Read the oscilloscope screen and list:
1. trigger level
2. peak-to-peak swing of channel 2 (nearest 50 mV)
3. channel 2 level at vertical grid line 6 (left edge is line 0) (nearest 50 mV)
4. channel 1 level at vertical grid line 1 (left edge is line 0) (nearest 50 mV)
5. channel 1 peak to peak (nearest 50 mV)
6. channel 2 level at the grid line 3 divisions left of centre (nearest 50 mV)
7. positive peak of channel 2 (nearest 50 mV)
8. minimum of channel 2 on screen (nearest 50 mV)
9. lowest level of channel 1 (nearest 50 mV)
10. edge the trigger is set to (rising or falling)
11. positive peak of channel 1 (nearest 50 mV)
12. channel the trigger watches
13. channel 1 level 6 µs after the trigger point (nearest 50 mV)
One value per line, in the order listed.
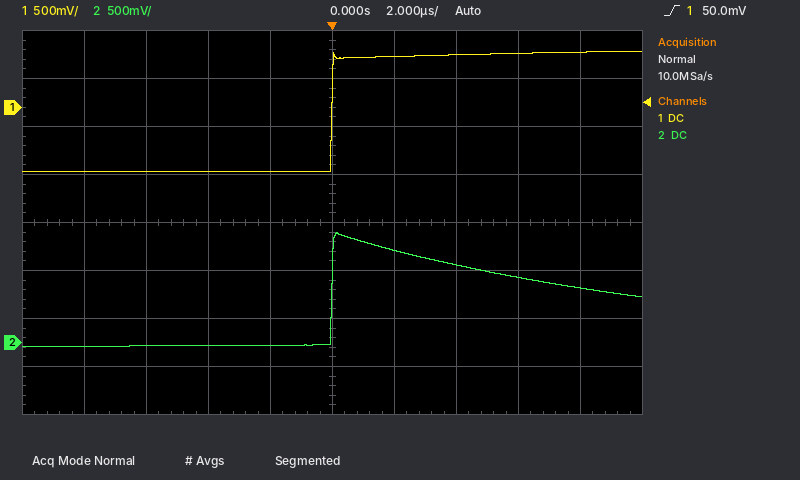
50.0 mV
1.20 V
950 mV
-650 mV
1.25 V
-50 mV
1.15 V
-50 mV
-650 mV
rising
600 mV
channel 1
550 mV
